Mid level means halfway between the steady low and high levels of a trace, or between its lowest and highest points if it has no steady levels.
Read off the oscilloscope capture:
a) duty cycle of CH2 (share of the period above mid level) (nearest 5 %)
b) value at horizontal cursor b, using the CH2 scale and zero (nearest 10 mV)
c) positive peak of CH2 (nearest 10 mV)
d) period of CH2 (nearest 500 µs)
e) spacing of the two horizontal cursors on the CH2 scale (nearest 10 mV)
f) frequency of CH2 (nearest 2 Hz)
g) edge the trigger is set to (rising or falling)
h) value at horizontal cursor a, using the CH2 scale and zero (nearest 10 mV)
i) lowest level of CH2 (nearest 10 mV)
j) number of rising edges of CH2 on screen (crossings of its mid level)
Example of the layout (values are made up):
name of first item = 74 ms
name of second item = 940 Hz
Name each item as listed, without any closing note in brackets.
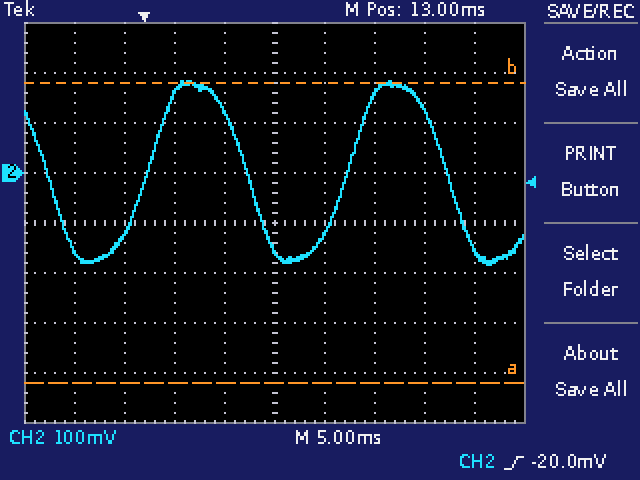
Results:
duty cycle of CH2 (share of the period above mid level) = 50 %
value at horizontal cursor b, using the CH2 scale and zero = 180 mV
positive peak of CH2 = 180 mV
period of CH2 = 20.0 ms
spacing of the two horizontal cursors on the CH2 scale = 600 mV
frequency of CH2 = 50 Hz
edge the trigger is set to = rising
value at horizontal cursor a, using the CH2 scale and zero = -420 mV
lowest level of CH2 = -180 mV
number of rising edges of CH2 on screen = 2
